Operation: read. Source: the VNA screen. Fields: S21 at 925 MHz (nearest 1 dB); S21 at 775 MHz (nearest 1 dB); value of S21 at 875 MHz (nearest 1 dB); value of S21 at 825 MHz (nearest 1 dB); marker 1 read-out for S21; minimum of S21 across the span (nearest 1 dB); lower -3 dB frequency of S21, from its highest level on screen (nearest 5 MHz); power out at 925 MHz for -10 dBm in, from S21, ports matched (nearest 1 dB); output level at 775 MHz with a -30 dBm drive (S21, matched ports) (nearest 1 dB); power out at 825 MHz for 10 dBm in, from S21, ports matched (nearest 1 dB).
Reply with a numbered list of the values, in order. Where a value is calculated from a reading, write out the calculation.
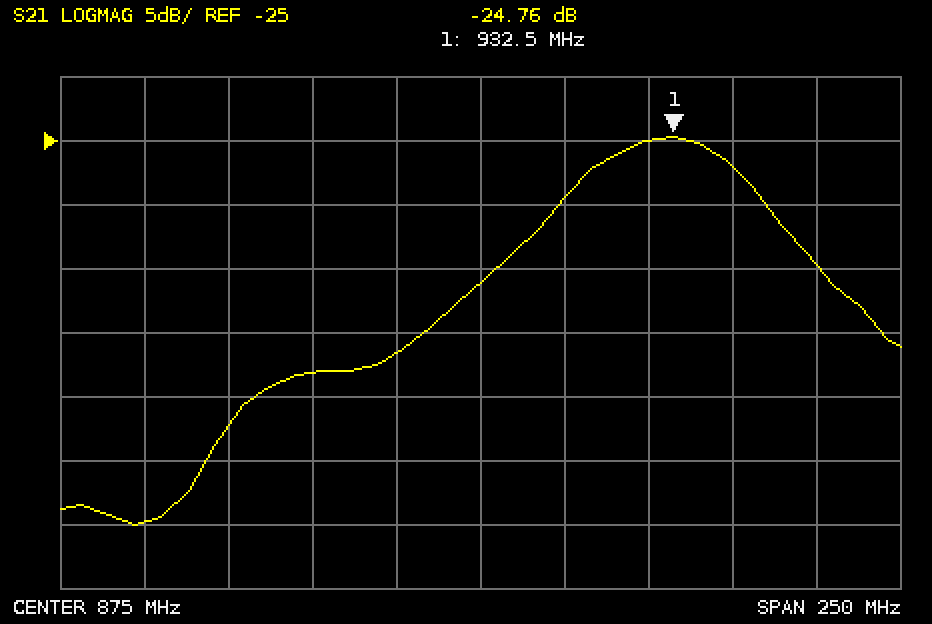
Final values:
1. -25 dB
2. -55 dB
3. -36 dB
4. -43 dB
5. -24.76 dB
6. -55 dB
7. 905 MHz
8. -10 dBm + (-25 dB) = -35 dBm
9. -30 dBm + (-55 dB) = -85 dBm
10. 10 dBm + (-43 dB) = -33 dBm
